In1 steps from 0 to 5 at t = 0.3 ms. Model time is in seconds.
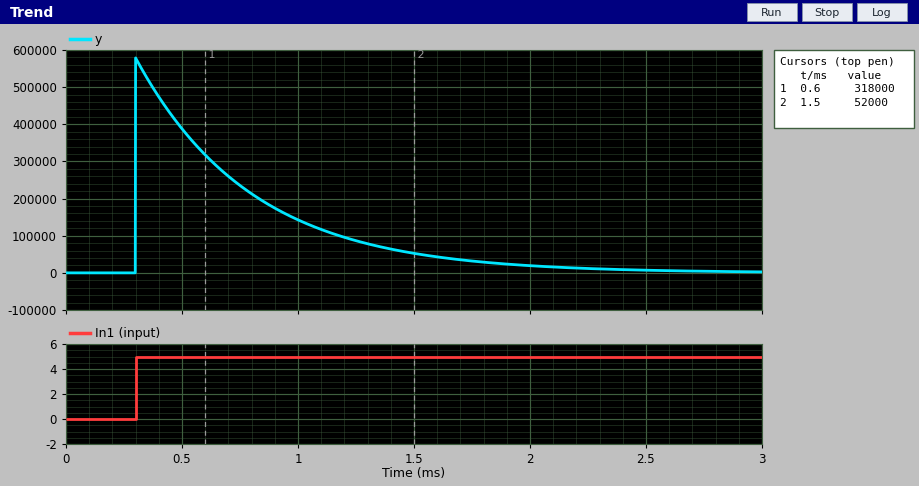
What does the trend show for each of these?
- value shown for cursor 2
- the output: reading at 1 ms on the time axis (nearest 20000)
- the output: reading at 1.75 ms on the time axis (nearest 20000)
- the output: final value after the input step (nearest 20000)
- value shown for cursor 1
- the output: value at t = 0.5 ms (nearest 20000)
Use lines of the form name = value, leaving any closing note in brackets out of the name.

value shown for cursor 2 = 52000
the output: reading at 1 ms on the time axis = 140000
the output: reading at 1.75 ms on the time axis = 40000
the output: final value after the input step = 0
value shown for cursor 1 = 318000
the output: value at t = 0.5 ms = 380000
